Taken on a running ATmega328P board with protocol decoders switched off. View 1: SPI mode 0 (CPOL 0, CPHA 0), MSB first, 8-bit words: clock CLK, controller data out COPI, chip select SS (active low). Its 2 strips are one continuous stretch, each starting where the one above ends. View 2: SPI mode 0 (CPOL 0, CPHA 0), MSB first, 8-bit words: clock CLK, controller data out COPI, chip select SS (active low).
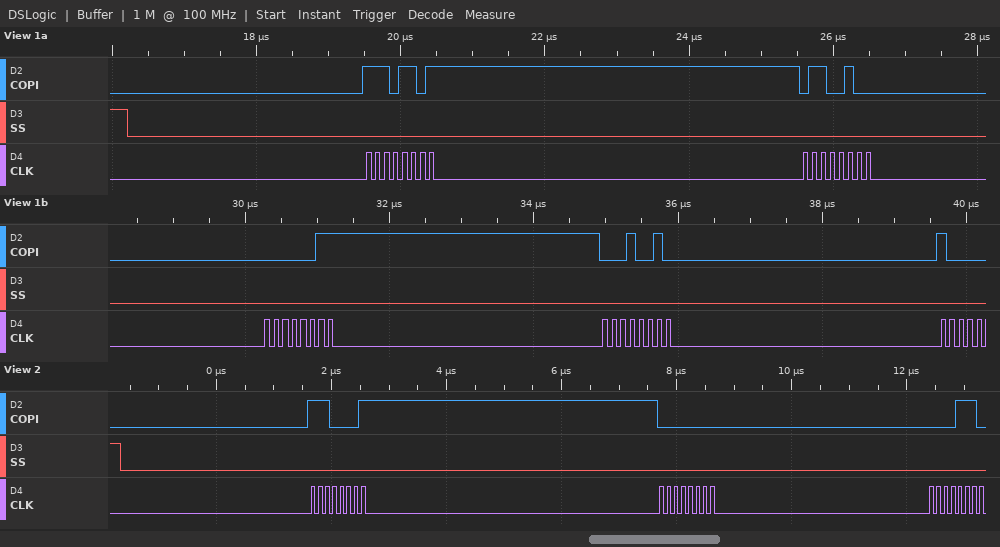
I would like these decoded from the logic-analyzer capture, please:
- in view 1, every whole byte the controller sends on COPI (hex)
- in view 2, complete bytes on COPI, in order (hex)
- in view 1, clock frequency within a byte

ED 64 03 12
0xE1 0x00 0x0E
8 MHz
